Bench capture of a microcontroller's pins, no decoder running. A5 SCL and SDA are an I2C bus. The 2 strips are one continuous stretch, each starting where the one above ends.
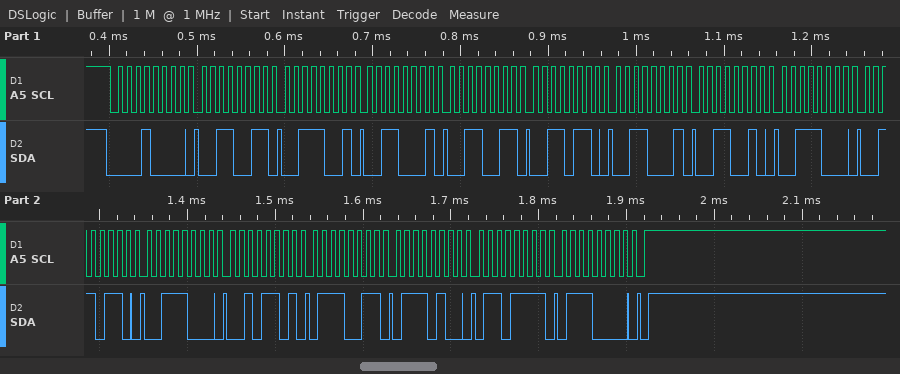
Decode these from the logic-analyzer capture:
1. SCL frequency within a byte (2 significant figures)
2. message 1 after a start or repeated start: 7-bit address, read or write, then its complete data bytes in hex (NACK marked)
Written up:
100 kHz
0x08 write: 33 39 31 33 36 31 32 38 36 38 2D 73 74 6F 70
